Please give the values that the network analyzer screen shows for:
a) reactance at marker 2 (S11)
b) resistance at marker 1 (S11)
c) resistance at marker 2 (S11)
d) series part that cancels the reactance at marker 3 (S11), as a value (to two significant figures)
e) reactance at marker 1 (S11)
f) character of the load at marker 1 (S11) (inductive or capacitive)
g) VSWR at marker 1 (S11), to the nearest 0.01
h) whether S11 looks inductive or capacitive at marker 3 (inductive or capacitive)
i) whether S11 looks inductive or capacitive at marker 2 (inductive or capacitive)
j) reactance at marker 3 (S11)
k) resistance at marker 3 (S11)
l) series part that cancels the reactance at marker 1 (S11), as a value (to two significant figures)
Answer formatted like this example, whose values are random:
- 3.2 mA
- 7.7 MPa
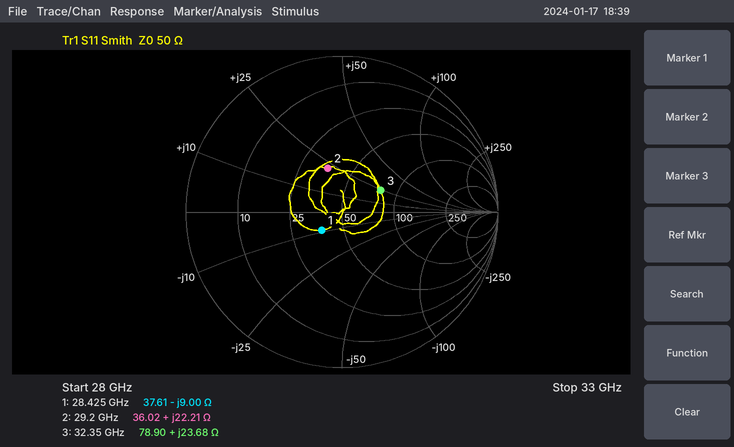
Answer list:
- +22.21 Ω
- 37.61 Ω
- 36.02 Ω
- 210 fF
- -9.00 Ω
- capacitive
- 1.42
- inductive
- inductive
- +23.68 Ω
- 78.90 Ω
- 50 pH
